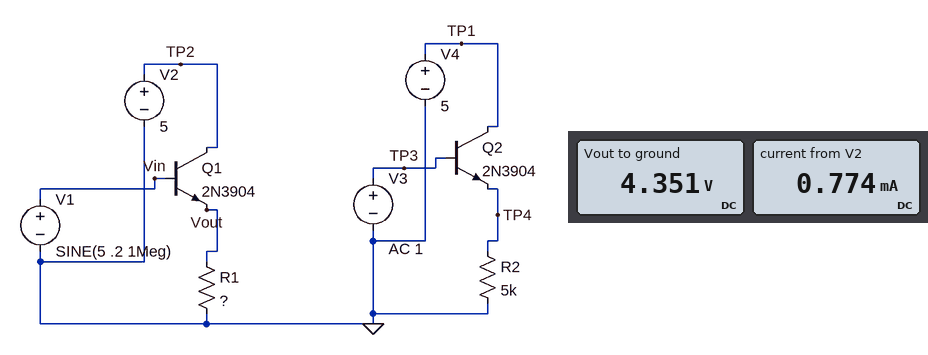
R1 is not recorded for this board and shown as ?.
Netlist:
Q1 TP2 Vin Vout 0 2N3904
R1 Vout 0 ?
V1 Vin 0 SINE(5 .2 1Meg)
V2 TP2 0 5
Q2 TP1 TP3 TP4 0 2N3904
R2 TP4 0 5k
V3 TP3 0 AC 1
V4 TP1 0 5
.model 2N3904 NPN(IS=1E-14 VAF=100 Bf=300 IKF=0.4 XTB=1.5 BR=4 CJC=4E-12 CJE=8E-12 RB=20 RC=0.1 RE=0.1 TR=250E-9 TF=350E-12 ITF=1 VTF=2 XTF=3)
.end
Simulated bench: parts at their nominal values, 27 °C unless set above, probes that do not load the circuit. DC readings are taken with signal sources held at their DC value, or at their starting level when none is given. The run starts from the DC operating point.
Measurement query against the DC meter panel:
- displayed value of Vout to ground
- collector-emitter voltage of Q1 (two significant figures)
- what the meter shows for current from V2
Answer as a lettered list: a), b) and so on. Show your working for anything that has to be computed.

a) 4.351 V
b) 5 V - 4.351 V = 650 mV
c) 0.774 mA
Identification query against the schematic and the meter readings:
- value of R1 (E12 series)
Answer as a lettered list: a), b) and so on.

a) 5.6 kΩ
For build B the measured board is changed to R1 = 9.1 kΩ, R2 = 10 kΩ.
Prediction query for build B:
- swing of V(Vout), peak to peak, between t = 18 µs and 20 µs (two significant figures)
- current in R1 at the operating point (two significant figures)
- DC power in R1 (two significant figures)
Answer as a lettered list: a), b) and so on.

a) 400 mV
b) 480 µA
c) 2.1 mW
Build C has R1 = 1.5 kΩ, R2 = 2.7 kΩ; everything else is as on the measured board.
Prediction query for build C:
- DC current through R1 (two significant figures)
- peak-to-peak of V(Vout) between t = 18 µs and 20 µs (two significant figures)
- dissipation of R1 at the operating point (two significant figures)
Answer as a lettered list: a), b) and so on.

a) 2.9 mA
b) 400 mV
c) 12 mW
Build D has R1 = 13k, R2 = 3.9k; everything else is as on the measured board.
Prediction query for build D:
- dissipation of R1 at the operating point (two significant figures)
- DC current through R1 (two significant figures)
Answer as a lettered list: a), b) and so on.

a) 1.5 mW
b) 340 µA
